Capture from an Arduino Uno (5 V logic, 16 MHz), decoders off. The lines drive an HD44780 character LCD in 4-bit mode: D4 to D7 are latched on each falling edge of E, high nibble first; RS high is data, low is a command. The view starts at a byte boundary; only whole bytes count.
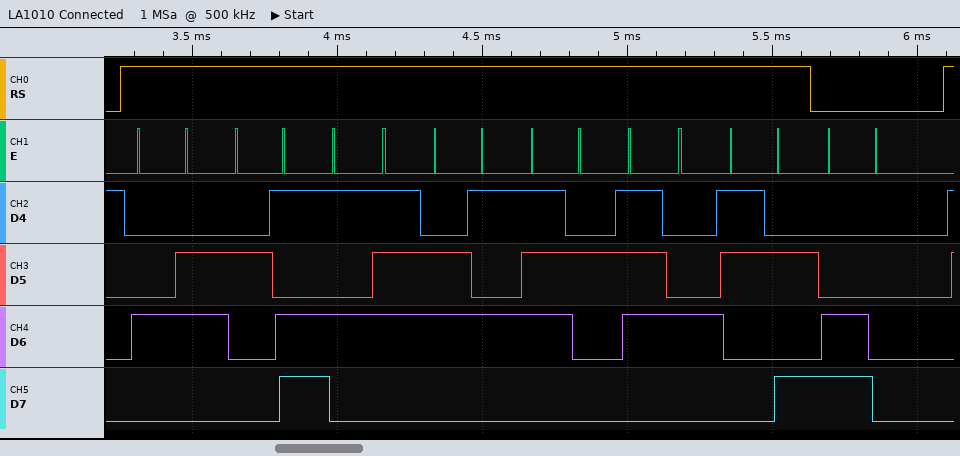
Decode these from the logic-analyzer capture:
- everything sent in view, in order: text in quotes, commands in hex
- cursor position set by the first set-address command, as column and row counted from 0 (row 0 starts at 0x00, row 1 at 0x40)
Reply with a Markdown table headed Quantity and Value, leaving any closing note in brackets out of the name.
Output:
| Quantity | Value |
|---|---|
| everything sent in view, in order: text in quotes, commands in hex | "F-Wert:" 0xC0 |
| cursor position set by the first set-address command, as column and row counted from 0 | column 0, row 1 |
